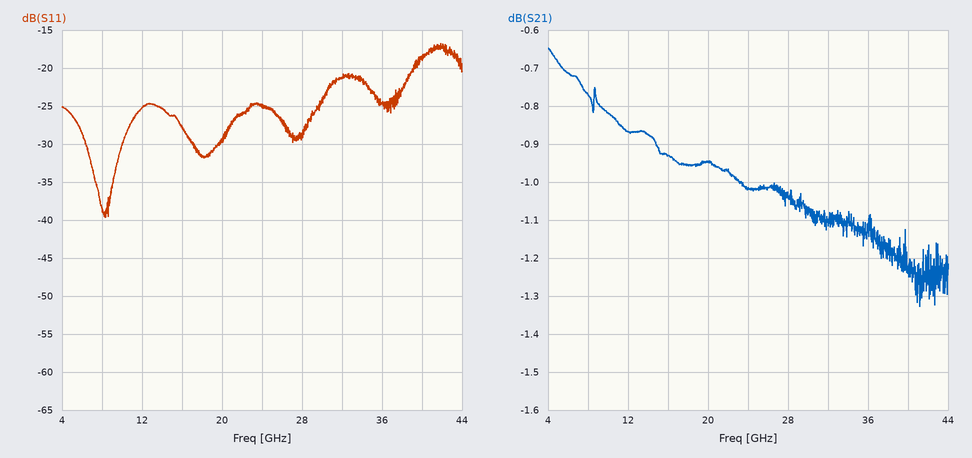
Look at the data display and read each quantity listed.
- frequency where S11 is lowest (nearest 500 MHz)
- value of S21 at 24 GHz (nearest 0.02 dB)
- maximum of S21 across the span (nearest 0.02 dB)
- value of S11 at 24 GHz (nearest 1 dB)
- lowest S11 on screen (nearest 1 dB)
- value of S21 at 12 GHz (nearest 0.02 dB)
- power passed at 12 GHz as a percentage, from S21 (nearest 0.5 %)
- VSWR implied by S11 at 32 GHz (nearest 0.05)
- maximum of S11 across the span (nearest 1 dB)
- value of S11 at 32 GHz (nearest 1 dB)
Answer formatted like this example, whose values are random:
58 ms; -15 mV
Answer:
8.5 GHz; -1.02 dB; -0.64 dB; -25 dB; -40 dB; -0.86 dB; 82.0 %; 1.20; -17 dB; -21 dB
